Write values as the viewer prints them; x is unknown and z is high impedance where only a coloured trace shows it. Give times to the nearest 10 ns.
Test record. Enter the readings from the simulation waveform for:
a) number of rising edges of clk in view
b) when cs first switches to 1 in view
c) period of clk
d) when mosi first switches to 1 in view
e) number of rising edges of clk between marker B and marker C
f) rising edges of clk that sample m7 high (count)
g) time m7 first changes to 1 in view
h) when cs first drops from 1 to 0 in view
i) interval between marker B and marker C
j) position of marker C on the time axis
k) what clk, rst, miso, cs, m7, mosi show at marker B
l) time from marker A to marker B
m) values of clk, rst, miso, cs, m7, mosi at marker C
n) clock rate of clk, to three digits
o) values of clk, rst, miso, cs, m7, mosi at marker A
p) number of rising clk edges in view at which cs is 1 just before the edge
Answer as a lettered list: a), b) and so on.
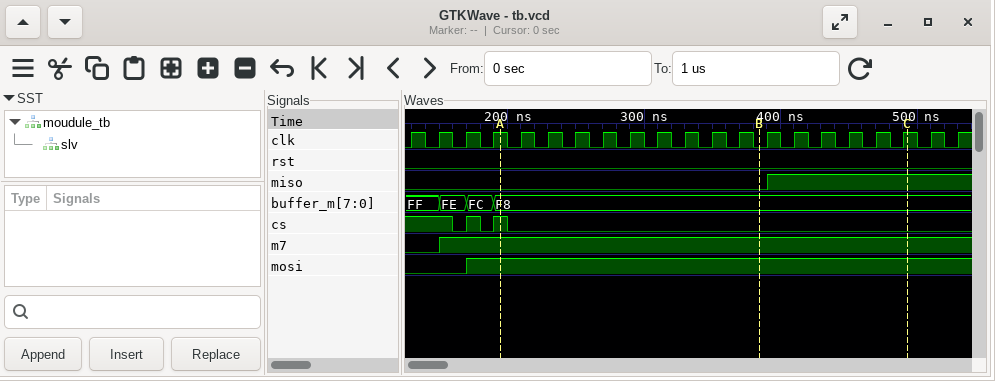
a) 21
b) 170 ns
c) 20 ns
d) 170 ns
e) 6
f) 19
g) 150 ns
h) 160 ns
i) 110 ns
j) 490 ns
k) clk=0, rst=0, miso=0, cs=0, m7=1, mosi=1
l) 190 ns
m) clk=1, rst=0, miso=1, cs=0, m7=1, mosi=1
n) 50.0 MHz
o) clk=1, rst=0, miso=0, cs=1, m7=1, mosi=1
p) 2
